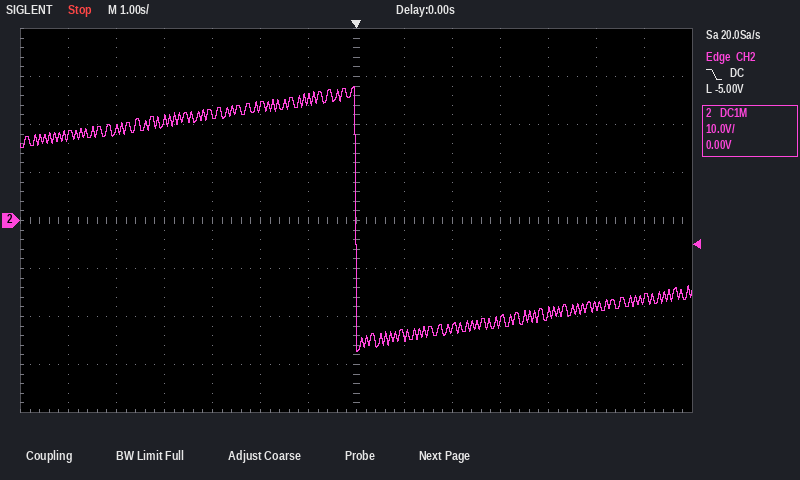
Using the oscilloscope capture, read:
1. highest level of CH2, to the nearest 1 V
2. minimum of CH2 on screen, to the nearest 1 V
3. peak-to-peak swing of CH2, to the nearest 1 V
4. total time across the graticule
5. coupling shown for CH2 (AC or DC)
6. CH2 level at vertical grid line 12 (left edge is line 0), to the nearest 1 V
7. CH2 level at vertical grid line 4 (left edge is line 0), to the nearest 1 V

28 V
-27 V
55 V
14 s
DC
-18 V
22 V
